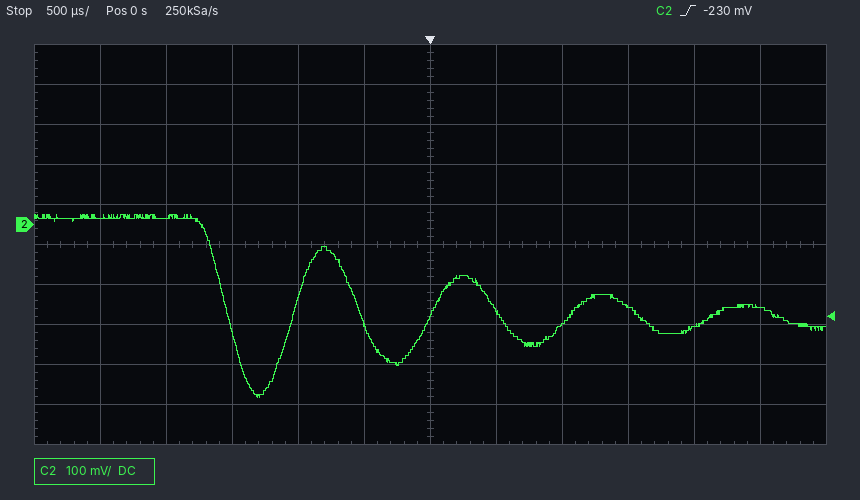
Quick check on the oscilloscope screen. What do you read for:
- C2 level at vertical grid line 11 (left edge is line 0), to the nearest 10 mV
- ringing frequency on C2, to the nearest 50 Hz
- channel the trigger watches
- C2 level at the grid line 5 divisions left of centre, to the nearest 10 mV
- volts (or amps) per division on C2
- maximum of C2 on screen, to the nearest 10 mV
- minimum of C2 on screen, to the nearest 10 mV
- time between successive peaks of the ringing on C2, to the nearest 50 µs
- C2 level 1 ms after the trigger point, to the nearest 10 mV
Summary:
-210 mV
950 Hz
C2
20 mV
100 mV
20 mV
-430 mV
1.05 ms
-250 mV
